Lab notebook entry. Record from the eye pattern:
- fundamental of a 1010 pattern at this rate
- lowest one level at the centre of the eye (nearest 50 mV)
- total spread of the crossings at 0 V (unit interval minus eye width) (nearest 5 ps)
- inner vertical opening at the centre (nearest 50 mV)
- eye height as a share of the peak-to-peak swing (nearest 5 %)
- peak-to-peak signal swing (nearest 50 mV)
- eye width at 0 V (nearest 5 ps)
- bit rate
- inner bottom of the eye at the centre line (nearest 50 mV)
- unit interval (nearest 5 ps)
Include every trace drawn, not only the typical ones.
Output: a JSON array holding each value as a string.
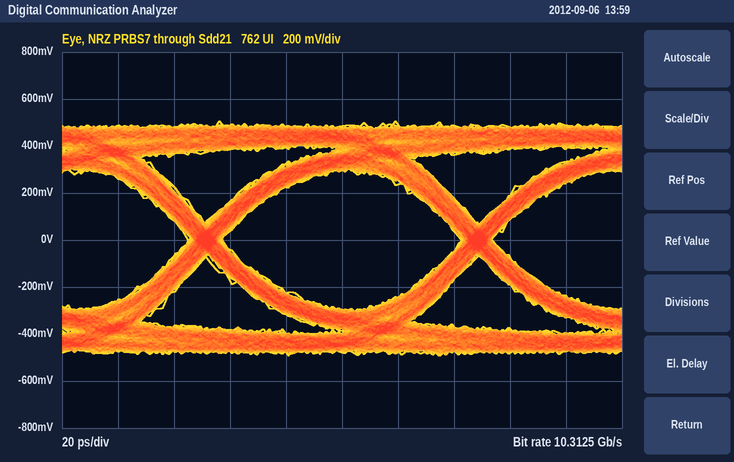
["5.15625 GHz", "300 mV", "10 ps", "600 mV", "60 %", "1.00 V", "85 ps", "10.3125 Gb/s", "-300 mV", "95 ps"]
